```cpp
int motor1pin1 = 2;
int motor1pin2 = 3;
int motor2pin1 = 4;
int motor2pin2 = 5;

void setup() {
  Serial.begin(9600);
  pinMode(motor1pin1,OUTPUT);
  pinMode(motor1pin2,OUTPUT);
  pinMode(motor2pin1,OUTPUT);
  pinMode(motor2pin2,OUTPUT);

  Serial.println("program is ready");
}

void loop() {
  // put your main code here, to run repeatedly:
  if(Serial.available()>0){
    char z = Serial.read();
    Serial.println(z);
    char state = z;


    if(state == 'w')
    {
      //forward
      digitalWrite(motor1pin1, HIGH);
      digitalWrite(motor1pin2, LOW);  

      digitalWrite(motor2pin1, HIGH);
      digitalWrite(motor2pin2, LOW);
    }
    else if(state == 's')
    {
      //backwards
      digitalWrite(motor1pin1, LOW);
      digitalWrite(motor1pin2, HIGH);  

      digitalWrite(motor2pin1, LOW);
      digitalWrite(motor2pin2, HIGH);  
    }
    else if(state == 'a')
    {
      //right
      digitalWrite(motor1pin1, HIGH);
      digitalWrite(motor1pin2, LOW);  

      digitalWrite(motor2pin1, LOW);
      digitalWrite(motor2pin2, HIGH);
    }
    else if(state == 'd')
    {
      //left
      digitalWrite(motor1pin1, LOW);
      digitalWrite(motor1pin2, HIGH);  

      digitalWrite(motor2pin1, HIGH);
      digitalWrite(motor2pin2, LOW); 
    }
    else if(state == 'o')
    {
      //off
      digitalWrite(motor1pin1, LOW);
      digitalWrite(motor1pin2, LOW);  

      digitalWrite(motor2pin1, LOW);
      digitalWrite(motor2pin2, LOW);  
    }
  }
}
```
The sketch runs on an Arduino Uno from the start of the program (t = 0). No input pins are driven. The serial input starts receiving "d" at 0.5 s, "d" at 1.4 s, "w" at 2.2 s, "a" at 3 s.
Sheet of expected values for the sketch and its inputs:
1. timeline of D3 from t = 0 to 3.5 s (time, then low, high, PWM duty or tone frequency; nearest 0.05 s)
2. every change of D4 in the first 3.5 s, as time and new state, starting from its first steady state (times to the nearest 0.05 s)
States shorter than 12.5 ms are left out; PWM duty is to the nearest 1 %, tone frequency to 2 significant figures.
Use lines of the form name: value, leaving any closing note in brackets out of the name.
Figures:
timeline of D3 from t = 0 to 3.5 s: 0 s low; 0.5 s high; 2.2 s low
every change of D4 in the first 3.5 s, as time and new state, starting from its first steady state: 0 s low; 0.5 s high; 3 s low
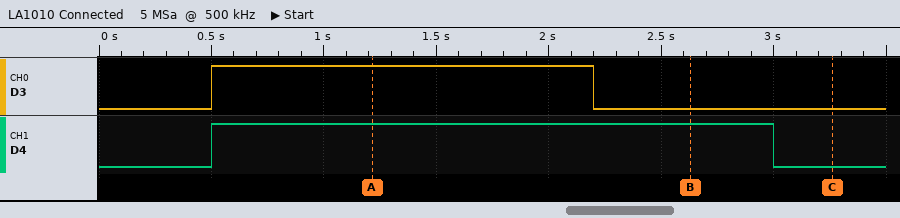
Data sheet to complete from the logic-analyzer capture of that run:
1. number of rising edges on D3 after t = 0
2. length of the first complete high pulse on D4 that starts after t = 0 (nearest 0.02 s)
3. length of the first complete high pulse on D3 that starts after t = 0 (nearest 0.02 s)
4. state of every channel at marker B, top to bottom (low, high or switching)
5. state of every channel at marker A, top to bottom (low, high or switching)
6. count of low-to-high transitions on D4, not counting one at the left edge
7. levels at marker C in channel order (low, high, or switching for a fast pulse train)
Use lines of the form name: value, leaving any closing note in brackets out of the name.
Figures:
number of rising edges on D3 after t = 0: 1
length of the first complete high pulse on D4 that starts after t = 0: 2.50 s
length of the first complete high pulse on D3 that starts after t = 0: 1.70 s
state of every channel at marker B, top to bottom: D3 low, D4 high
state of every channel at marker A, top to bottom: D3 high, D4 high
count of low-to-high transitions on D4, not counting one at the left edge: 1
levels at marker C in channel order: D3 low, D4 low
